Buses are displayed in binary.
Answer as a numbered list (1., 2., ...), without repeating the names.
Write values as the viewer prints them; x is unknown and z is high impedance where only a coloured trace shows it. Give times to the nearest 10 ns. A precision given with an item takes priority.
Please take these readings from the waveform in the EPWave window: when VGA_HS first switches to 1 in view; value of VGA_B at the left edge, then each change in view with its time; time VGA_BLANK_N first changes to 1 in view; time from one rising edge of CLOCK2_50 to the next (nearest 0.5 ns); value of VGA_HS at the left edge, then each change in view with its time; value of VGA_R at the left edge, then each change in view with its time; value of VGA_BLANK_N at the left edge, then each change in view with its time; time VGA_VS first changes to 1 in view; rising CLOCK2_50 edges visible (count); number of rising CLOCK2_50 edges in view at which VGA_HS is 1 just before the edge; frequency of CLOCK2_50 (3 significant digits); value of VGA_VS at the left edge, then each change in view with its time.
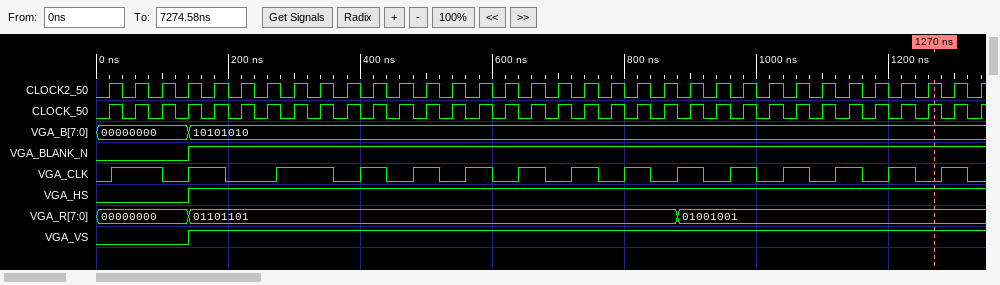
1. 140 ns
2. 00000000, 10101010 at 140 ns
3. 140 ns
4. 40 ns
5. 0, 1 at 140 ns
6. 00000000, 01101101 at 140 ns, 01001001 at 880 ns
7. 0, 1 at 140 ns
8. 140 ns
9. 34
10. 30
11. 25.0 MHz
12. 0, 1 at 140 ns
